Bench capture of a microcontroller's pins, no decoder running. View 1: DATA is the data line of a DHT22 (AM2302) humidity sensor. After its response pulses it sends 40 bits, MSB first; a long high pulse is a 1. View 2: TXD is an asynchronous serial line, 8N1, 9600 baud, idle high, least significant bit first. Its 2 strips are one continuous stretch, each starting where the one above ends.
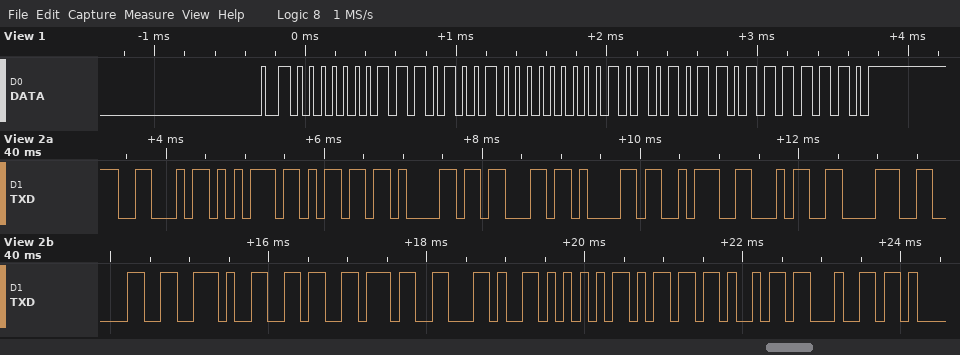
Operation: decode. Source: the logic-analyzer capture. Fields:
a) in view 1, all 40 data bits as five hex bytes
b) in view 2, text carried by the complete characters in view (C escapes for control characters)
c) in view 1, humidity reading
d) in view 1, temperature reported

01 D2 00 AB 7E
"Fumaca:480.67,Umid"
46.6 %
17.1 °C
